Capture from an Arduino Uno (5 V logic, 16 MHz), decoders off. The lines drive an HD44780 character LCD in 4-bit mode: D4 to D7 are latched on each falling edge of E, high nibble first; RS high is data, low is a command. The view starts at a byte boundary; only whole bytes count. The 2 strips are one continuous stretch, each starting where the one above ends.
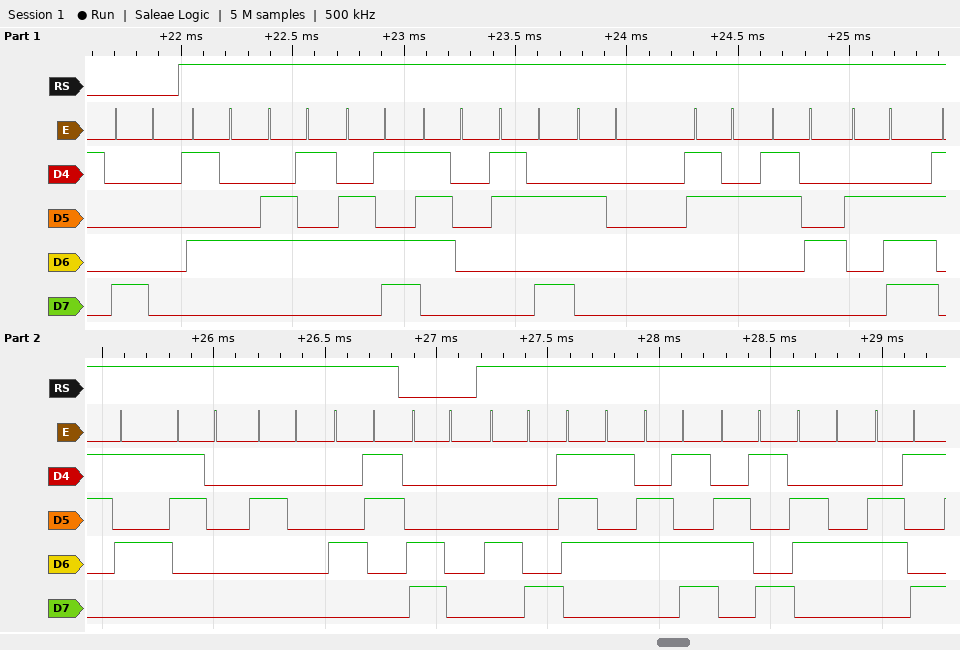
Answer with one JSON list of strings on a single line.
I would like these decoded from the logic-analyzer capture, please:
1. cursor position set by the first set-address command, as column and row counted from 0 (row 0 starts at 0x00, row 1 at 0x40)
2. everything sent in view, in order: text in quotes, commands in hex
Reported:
["column 0, row 0", "0x80 \"Temp: 24.50 C\" 0xC0 \"Humidi\""]
